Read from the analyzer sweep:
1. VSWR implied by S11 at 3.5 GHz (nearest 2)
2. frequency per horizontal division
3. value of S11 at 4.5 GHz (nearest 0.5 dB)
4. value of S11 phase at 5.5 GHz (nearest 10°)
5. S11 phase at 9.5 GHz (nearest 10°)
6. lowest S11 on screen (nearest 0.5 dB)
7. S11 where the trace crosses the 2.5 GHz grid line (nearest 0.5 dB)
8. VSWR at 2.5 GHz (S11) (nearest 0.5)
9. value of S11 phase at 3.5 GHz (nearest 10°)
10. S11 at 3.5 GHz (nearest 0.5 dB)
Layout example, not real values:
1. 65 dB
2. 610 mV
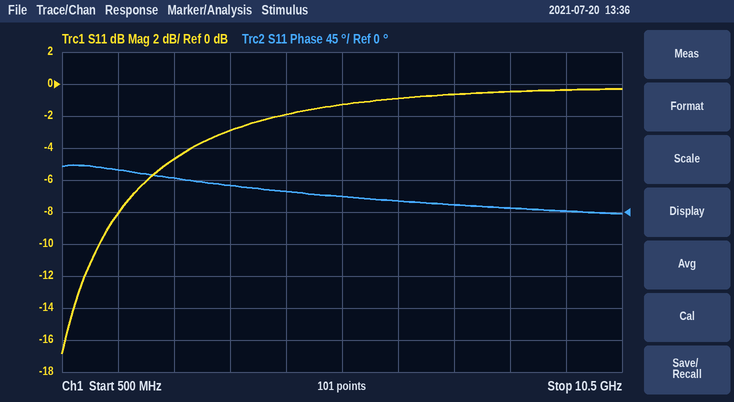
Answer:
1. 6
2. 1 GHz
3. -2.0 dB
4. 20°
5. 0°
6. -17.0 dB
7. -4.5 dB
8. 4.0
9. 40°
10. -3.0 dB
